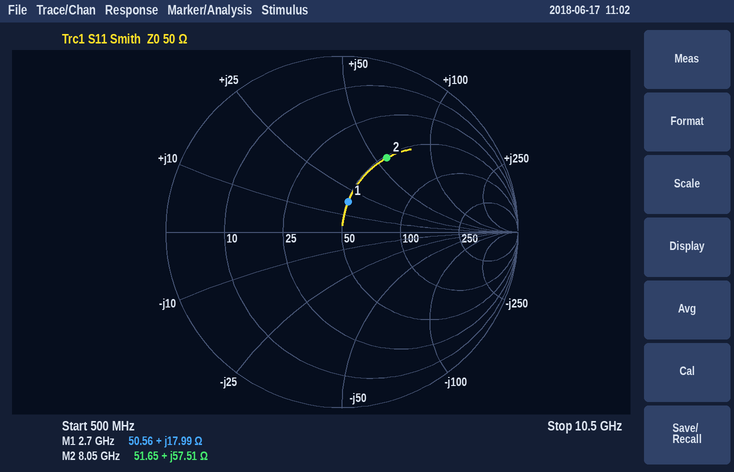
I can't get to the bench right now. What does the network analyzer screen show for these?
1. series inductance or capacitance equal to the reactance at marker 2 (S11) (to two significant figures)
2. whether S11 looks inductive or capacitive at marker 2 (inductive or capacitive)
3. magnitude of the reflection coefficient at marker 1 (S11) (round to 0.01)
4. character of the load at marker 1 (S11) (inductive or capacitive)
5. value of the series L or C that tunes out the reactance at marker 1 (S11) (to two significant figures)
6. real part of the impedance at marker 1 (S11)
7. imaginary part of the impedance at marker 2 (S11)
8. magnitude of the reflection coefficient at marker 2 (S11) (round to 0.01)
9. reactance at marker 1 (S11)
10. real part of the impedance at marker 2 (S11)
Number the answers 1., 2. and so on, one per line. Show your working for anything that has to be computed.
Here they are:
1. L = 57.51 Ω/(2π × 8.05 GHz) ≈ 1.1 nH
2. inductive
3. 0.18
4. inductive
5. C = 1/(2π × 2.7 GHz × 17.99 Ω) ≈ 3.3 pF
6. 50.56 Ω
7. +57.51 Ω
8. 0.49
9. +17.99 Ω
10. 51.65 Ω
